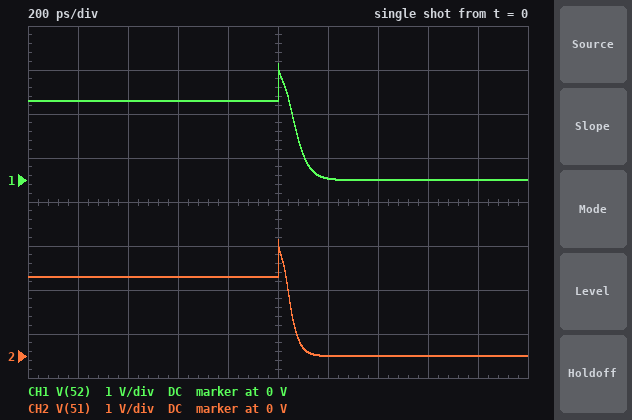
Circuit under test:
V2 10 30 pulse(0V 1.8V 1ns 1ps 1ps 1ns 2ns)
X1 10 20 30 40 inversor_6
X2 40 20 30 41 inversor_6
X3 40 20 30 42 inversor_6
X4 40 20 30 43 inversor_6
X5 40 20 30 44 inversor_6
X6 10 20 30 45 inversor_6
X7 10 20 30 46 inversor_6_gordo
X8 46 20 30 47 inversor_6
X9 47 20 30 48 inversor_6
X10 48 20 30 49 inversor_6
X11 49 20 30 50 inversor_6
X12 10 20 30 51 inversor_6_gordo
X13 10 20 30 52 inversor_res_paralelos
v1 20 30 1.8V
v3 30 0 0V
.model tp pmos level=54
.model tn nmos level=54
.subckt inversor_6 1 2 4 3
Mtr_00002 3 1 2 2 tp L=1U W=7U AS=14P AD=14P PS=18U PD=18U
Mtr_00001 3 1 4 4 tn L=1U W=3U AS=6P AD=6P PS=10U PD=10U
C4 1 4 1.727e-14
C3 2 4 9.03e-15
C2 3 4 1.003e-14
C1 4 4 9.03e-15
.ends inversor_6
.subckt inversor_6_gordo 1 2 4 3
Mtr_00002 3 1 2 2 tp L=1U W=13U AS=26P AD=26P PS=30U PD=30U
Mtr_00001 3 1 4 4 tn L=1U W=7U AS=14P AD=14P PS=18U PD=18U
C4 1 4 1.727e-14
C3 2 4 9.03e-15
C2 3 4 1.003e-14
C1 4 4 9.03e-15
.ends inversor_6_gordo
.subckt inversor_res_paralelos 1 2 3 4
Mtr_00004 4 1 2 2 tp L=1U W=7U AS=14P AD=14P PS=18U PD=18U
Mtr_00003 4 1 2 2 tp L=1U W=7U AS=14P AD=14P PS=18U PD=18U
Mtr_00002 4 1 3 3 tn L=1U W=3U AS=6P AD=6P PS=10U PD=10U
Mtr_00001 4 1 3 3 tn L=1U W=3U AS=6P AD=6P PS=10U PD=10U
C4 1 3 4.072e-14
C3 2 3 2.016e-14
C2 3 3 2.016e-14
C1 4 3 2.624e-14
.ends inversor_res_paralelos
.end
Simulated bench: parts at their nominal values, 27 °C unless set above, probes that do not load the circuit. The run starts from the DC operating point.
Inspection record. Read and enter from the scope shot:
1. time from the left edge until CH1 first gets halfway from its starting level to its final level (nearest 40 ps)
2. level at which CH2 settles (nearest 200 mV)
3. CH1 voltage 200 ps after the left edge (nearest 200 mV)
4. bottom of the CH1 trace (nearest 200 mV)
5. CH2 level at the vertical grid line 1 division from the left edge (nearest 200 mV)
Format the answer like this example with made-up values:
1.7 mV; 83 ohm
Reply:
1.08 ns; 0 V; 1.8 V; 0 V; 1.8 V
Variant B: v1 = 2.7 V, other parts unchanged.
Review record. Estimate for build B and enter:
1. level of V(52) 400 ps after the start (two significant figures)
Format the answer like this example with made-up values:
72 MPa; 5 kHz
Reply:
2.7 V
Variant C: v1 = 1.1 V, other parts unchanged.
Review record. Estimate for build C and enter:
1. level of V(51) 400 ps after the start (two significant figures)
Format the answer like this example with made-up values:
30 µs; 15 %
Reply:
1.1 V
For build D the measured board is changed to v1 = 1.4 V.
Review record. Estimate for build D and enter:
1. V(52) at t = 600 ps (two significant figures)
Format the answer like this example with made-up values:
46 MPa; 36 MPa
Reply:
1.4 V
